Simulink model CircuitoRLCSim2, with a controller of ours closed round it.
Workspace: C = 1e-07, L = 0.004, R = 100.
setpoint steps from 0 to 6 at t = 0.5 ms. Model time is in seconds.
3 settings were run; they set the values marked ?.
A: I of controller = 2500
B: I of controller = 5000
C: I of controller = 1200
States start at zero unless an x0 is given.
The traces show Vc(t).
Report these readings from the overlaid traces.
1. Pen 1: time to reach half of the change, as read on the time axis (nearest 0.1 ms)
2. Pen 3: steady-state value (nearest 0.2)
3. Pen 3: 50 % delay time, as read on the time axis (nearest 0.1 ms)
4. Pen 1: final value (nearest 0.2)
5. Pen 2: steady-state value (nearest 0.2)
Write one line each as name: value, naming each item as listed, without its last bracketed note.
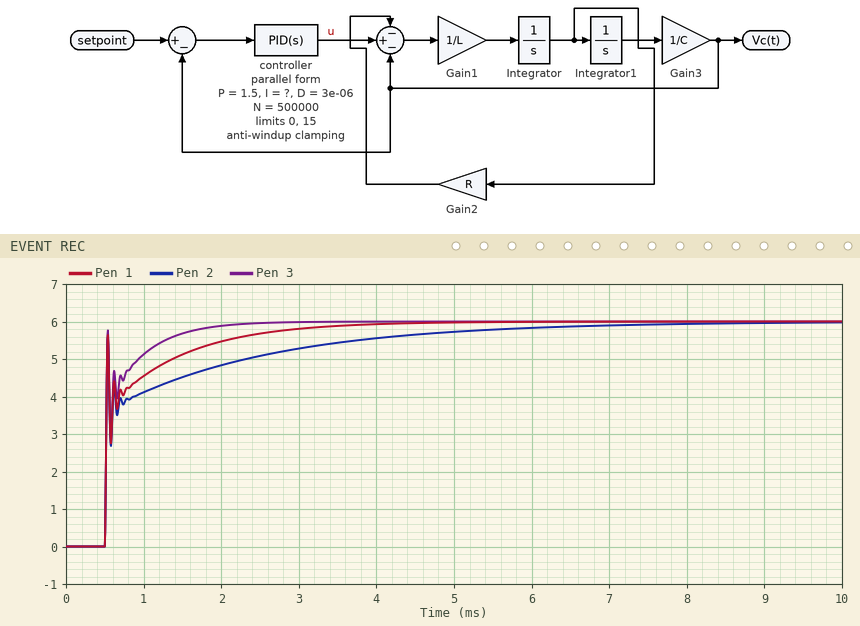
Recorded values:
Pen 1: time to reach half of the change, as read on the time axis: 0.5 ms
Pen 3: steady-state value: 6.0
Pen 3: 50 % delay time, as read on the time axis: 0.5 ms
Pen 1: final value: 6.0
Pen 2: steady-state value: 6.0
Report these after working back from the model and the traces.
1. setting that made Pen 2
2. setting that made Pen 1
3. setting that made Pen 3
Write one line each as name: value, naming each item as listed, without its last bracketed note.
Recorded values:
setting that made Pen 2: C
setting that made Pen 1: A
setting that made Pen 3: B
